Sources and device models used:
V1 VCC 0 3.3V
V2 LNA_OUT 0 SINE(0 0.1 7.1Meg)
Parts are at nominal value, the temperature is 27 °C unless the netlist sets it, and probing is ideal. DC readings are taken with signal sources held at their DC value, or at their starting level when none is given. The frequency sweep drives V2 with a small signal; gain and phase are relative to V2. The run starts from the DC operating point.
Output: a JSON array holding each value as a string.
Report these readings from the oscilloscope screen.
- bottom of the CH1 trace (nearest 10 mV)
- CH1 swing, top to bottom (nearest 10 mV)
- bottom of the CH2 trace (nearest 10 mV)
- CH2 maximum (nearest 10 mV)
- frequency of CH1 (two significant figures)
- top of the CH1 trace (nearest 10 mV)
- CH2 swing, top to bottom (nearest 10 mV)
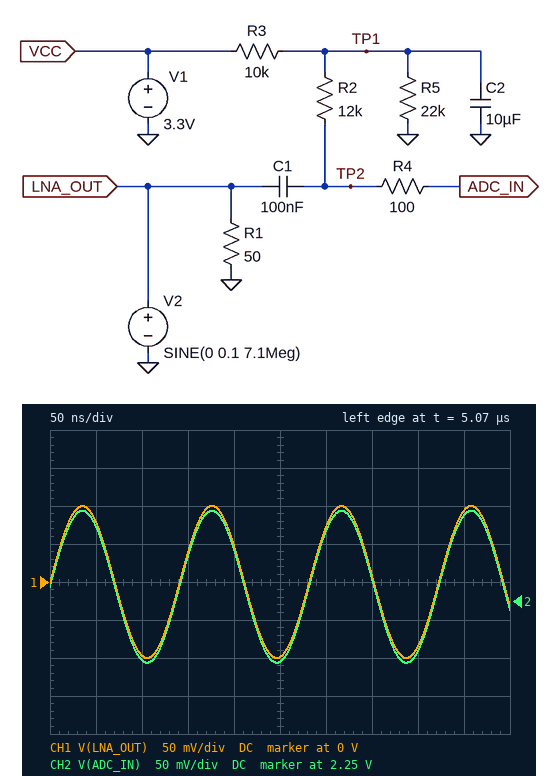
["-100 mV", "200 mV", "2.17 V", "2.37 V", "7.1 MHz", "100 mV", "200 mV"]
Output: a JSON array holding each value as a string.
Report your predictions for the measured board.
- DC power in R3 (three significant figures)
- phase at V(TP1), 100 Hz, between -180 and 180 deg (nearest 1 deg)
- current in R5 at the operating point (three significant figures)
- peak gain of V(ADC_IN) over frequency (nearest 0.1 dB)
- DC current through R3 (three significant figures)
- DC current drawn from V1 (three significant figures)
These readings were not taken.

["106 µW", "-35 deg", "103 µA", "0 dB", "103 µA", "103 µA"]
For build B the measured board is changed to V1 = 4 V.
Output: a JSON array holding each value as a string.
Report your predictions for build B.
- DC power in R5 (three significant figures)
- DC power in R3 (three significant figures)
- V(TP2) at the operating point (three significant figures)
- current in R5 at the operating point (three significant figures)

["344 µW", "156 µW", "2.75 V", "125 µA"]
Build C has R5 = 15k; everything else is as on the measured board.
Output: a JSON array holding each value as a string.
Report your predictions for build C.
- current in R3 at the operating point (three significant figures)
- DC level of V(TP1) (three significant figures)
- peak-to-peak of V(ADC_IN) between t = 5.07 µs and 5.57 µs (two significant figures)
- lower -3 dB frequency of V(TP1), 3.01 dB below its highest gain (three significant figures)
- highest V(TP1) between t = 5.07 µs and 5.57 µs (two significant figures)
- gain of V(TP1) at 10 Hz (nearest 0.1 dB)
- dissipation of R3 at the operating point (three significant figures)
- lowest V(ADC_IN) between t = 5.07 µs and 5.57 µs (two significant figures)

["132 µA", "1.98 V", "200 mV", "2.53 Hz", "2.0 V", "-40.4 dB", "174 µW", "1.9 V"]
